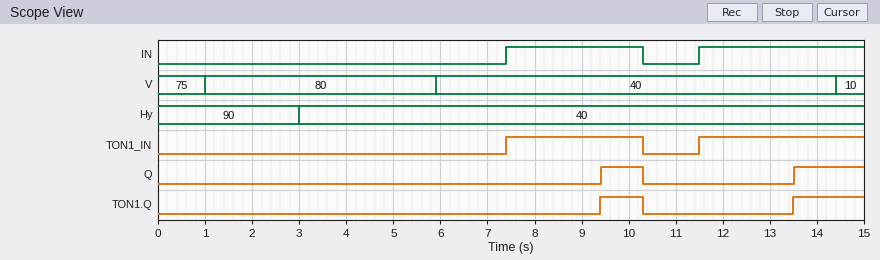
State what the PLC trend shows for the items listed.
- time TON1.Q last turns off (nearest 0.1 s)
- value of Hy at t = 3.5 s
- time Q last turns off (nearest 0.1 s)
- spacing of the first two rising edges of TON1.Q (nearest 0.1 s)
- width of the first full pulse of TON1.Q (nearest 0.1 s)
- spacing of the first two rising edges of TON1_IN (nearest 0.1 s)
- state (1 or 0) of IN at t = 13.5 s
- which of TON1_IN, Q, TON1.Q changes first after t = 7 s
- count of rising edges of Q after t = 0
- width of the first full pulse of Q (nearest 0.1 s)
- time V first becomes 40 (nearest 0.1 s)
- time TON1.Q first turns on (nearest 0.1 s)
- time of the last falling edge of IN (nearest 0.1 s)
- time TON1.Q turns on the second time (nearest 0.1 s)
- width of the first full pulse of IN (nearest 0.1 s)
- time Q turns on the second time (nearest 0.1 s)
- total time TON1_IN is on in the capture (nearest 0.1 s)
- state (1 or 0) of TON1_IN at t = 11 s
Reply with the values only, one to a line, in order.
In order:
10.3 s
40
10.3 s
4.1 s
0.9 s
4.1 s
1
TON1_IN
2
0.9 s
5.9 s
9.4 s
10.3 s
13.5 s
2.9 s
13.5 s
6.4 s
0
